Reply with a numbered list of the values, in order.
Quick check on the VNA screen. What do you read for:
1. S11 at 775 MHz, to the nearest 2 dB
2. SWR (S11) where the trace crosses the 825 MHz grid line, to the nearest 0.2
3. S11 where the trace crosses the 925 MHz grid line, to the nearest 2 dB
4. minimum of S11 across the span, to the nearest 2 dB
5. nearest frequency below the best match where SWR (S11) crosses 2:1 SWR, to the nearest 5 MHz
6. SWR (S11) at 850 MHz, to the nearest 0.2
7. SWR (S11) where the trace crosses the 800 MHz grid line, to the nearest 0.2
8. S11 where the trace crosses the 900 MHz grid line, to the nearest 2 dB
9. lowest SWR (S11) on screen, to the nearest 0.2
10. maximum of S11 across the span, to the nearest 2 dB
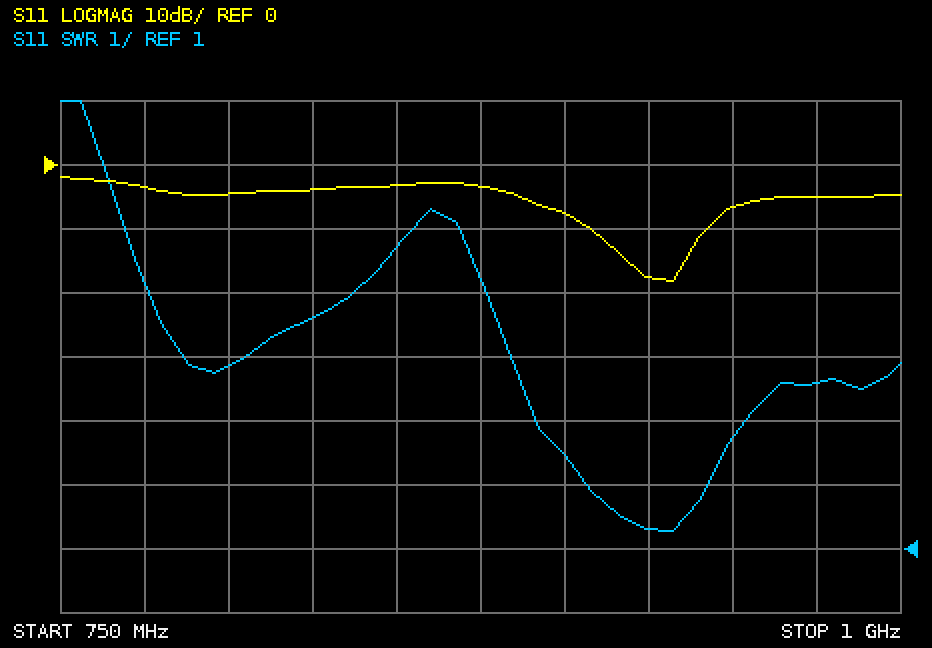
1. -4 dB
2. 4.6
3. -18 dB
4. -18 dB
5. 905 MHz
6. 5.8
7. 3.8
8. -8 dB
9. 1.2
10. -2 dB
